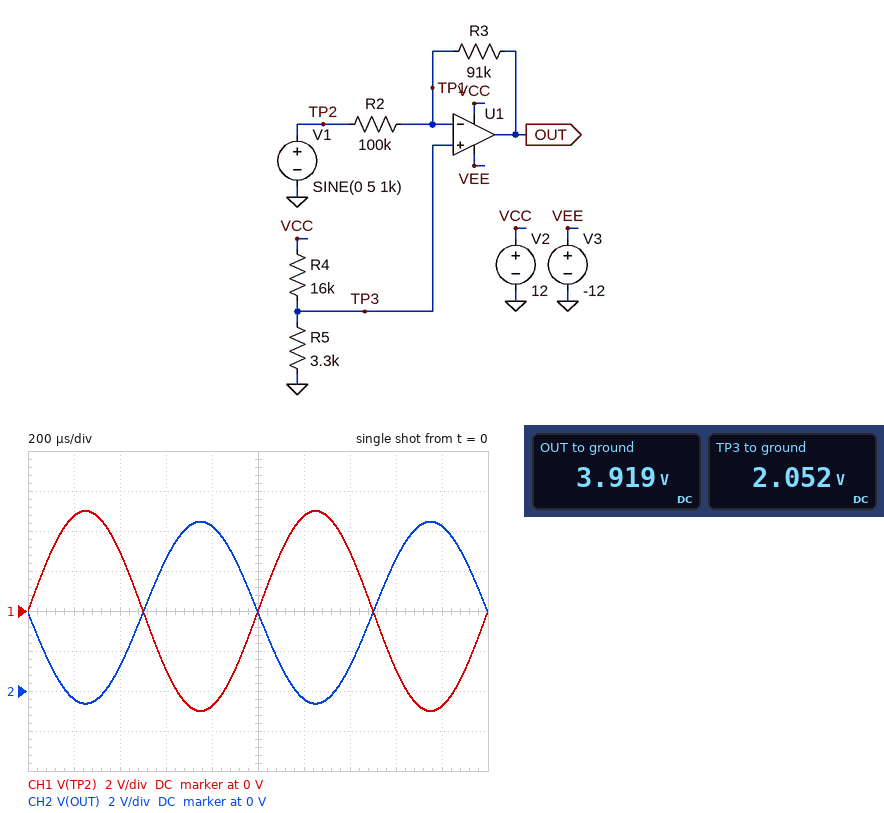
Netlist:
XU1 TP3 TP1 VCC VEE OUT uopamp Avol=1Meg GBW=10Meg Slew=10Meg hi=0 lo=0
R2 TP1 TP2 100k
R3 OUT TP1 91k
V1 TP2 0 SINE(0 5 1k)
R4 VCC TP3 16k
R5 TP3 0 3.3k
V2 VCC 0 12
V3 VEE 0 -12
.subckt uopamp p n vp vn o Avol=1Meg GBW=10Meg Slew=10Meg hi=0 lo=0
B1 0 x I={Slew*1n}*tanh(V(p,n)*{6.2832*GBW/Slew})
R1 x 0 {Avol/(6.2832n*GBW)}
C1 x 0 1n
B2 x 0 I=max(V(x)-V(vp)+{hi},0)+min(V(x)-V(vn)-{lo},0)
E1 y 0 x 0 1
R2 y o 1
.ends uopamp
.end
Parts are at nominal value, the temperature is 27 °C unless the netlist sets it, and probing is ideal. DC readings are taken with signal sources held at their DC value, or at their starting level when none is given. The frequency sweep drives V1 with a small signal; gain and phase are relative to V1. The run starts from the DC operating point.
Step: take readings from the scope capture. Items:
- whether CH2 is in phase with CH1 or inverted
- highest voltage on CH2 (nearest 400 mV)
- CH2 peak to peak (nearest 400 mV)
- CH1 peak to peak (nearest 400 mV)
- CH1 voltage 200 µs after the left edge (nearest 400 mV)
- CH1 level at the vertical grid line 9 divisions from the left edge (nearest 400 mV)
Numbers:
inverted
8.4 V
9.2 V
10.0 V
4.8 V
-4.8 V
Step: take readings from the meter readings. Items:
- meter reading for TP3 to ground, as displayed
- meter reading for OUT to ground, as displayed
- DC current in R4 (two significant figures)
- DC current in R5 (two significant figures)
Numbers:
2.052 V
3.919 V
620 µA
620 µA
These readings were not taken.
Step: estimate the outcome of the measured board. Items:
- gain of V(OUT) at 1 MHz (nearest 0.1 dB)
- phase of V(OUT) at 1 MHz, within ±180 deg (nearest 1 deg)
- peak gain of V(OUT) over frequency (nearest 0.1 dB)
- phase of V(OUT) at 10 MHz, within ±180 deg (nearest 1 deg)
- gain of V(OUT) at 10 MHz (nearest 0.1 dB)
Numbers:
-1.0 dB
169 deg
-0.8 dB
118 deg
-7.5 dB
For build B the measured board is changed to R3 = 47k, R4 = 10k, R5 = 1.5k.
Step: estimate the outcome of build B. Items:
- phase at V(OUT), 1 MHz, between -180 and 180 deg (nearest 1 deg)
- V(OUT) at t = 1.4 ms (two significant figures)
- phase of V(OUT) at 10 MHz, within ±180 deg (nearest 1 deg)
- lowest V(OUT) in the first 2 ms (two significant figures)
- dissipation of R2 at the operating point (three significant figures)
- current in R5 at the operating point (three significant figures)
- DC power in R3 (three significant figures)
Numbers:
172 deg
920 mV
124 deg
-49 mV
24.5 µW
1.04 mA
11.5 µW
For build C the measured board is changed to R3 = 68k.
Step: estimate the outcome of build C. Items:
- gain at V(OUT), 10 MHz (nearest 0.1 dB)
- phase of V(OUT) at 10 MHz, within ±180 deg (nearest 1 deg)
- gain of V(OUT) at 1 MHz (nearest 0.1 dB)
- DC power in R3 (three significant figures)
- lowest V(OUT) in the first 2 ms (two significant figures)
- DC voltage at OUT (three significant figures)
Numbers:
-9.2 dB
121 deg
-3.5 dB
28.6 µW
47 mV
3.45 V
